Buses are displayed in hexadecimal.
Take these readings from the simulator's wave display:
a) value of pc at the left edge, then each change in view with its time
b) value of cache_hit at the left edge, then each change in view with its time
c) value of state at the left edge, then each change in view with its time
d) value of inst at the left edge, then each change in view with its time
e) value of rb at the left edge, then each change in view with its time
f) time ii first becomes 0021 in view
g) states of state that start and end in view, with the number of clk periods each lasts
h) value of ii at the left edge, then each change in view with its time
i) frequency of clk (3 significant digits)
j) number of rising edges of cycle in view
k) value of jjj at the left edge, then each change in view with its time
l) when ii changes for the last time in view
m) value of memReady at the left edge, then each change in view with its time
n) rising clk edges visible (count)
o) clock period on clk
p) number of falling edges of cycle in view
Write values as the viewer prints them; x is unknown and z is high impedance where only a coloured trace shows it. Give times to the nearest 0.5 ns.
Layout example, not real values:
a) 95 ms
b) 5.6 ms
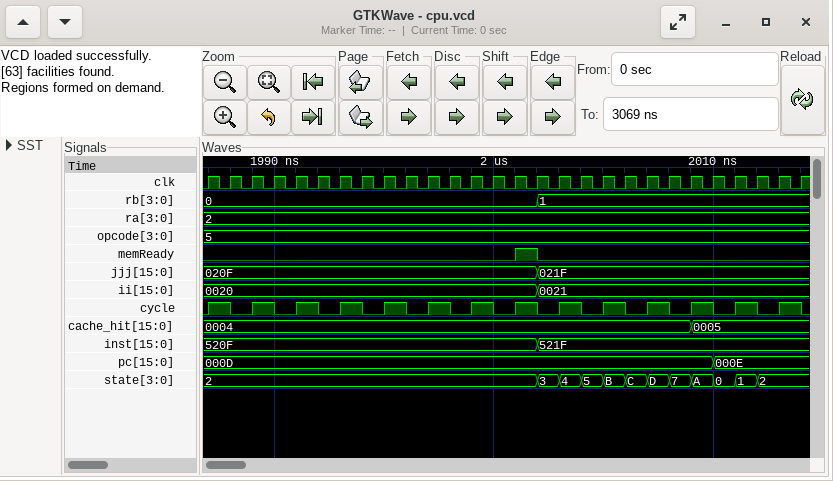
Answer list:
a) 000D, 000E at 2010 ns
b) 0004, 0005 at 2009 ns
c) 2, 3 at 2002 ns, 4 at 2003 ns, 5 at 2004 ns, B at 2005 ns, C at 2006 ns, D at 2007 ns, 7 at 2008 ns, A at 2009 ns, 0 at 2010 ns, 1 at 2011 ns, 2 at 2012 ns
d) 520F, 521F at 2002 ns
e) 0, 1 at 2002 ns
f) 2002 ns
g) 3: 1, 4: 1, 5: 1, B: 1, C: 1, D: 1, 7: 1, A: 1, 0: 1, 1: 1
h) 0020, 0021 at 2002 ns
i) 1.00 GHz
j) 14
k) 020F, 021F at 2002 ns
l) 2002 ns
m) 0, 1 at 2001 ns, 0 at 2002 ns
n) 28
o) 1 ns
p) 14
